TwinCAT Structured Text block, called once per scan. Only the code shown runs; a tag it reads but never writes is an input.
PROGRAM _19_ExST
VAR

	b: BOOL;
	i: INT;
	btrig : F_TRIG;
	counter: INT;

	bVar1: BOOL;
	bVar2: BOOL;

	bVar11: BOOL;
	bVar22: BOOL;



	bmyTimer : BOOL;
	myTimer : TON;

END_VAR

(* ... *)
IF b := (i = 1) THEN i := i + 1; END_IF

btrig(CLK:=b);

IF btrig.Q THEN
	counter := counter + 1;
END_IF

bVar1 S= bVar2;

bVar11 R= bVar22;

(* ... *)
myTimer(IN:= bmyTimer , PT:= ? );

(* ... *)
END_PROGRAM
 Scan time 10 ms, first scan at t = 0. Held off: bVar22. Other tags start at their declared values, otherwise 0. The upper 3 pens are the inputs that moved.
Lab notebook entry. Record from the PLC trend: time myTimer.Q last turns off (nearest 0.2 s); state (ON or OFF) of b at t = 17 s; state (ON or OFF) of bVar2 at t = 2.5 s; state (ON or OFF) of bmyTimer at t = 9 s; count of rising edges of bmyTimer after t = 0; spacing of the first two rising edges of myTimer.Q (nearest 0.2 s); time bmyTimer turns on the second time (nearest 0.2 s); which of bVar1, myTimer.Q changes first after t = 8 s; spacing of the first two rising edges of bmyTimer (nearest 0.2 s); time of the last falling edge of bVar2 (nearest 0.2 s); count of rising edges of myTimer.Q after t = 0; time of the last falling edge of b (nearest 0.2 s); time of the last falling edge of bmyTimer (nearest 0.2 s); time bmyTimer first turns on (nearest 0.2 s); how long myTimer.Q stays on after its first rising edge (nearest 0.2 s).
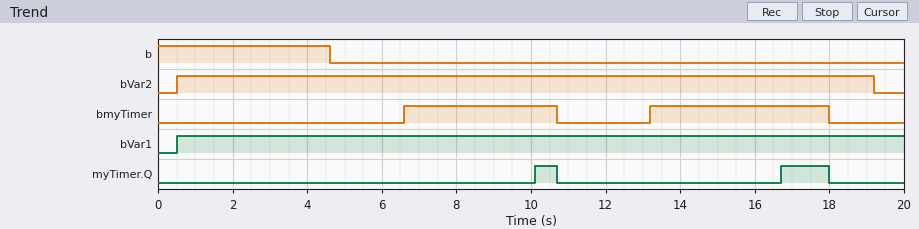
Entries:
18.0 s
OFF
ON
ON
2
6.6 s
13.2 s
myTimer.Q
6.6 s
19.2 s
2
4.6 s
18.0 s
6.6 s
0.6 s
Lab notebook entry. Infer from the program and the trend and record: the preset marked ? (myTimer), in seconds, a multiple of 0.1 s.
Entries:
3.5 s
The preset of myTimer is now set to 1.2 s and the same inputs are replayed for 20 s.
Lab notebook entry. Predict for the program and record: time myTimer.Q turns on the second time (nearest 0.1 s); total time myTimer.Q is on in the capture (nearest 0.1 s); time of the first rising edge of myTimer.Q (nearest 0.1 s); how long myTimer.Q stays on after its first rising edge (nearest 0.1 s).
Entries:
14.4 s
6.5 s
7.8 s
2.9 s
